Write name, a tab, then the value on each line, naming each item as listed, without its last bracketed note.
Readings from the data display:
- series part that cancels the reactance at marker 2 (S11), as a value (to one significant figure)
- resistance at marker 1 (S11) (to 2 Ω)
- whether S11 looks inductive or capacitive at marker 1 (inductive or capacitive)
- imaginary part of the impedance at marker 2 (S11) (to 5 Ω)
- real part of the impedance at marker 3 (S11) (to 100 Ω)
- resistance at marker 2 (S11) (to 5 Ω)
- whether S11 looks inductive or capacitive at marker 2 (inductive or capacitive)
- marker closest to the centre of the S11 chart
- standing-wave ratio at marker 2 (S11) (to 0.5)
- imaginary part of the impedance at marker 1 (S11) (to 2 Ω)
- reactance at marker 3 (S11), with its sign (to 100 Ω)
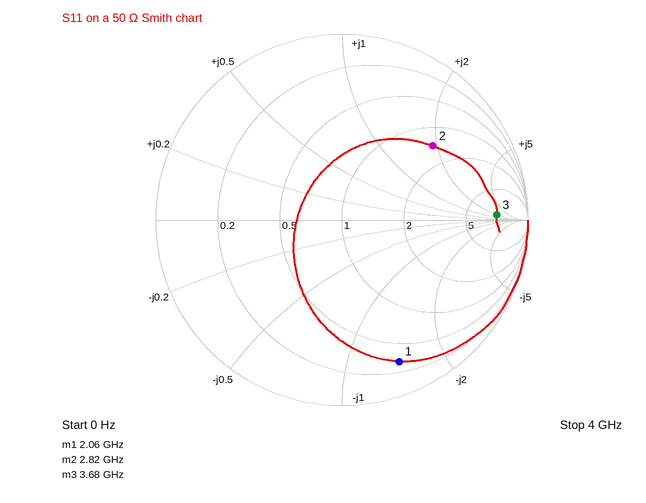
series part that cancels the reactance at marker 2 (S11), as a value	600 fF
resistance at marker 1 (S11)	16 Ω
whether S11 looks inductive or capacitive at marker 1	capacitive
imaginary part of the impedance at marker 2 (S11)	+95 Ω
real part of the impedance at marker 3 (S11)	500 Ω
resistance at marker 2 (S11)	70 Ω
whether S11 looks inductive or capacitive at marker 2	inductive
marker closest to the centre of the S11 chart	marker 2
standing-wave ratio at marker 2 (S11)	4.5
imaginary part of the impedance at marker 1 (S11)	-72 Ω
reactance at marker 3 (S11), with its sign	+100 Ω
